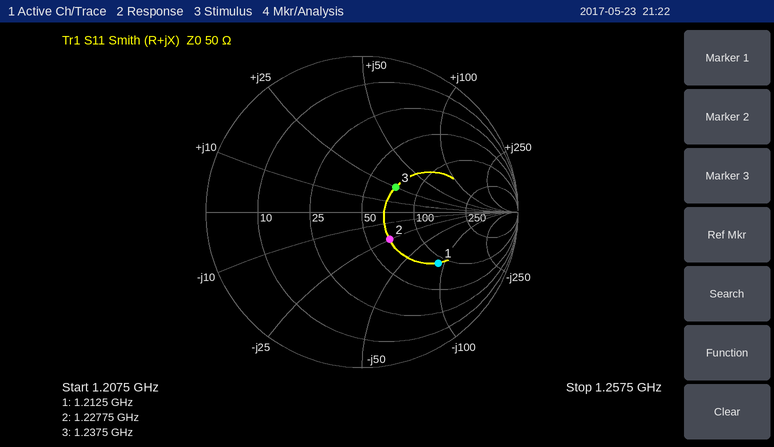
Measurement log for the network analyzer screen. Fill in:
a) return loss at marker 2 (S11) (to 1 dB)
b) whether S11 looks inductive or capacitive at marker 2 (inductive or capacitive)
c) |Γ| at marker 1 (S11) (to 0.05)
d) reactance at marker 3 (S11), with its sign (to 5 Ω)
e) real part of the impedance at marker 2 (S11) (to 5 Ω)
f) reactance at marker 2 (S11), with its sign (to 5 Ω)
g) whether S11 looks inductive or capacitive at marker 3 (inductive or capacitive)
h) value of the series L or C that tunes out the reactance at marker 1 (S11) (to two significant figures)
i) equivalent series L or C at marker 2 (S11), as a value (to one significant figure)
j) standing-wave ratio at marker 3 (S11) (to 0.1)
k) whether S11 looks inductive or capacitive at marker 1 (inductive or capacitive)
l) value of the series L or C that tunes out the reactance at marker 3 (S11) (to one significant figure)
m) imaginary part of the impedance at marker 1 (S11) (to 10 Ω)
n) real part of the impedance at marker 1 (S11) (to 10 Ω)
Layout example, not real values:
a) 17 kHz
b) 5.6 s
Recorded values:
a) 12 dB
b) capacitive
c) 0.60
d) +25 Ω
e) 65 Ω
f) -25 Ω
g) inductive
h) 12 nH
i) 5 pF
j) 1.7
k) capacitive
l) 5 pF
m) -90 Ω
n) 90 Ω
